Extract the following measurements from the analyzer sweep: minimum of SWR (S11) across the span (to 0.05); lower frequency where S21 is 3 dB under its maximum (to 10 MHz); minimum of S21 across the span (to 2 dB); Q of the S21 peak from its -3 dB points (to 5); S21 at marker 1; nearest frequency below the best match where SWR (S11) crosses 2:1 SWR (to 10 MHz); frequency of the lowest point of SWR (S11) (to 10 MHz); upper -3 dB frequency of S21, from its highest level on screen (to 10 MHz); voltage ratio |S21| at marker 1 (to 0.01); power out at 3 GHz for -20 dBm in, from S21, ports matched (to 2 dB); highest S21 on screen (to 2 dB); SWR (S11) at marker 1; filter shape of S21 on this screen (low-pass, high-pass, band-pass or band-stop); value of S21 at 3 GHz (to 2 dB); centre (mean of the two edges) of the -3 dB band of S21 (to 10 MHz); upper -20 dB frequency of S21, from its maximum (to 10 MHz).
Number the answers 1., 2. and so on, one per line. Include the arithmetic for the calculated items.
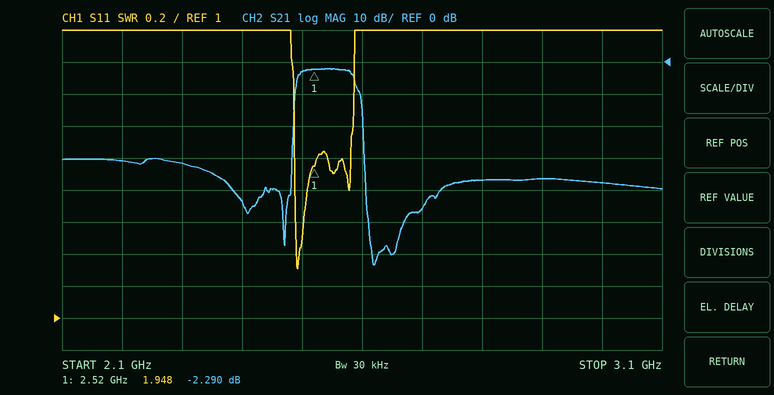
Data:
1. 1.30
2. 2.49 GHz
3. -64 dB
4. 2.54 GHz / 100 MHz ≈ 25
5. -2.290 dB
6. 2.49 GHz
7. 2.49 GHz
8. 2.59 GHz
9. 10^(-2.29/20) ≈ 0.77
10. -20 dBm + (-38 dB) = -58 dBm
11. -2 dB
12. 1.948
13. band-pass
14. -38 dB
15. 2.54 GHz
16. 2.60 GHz
